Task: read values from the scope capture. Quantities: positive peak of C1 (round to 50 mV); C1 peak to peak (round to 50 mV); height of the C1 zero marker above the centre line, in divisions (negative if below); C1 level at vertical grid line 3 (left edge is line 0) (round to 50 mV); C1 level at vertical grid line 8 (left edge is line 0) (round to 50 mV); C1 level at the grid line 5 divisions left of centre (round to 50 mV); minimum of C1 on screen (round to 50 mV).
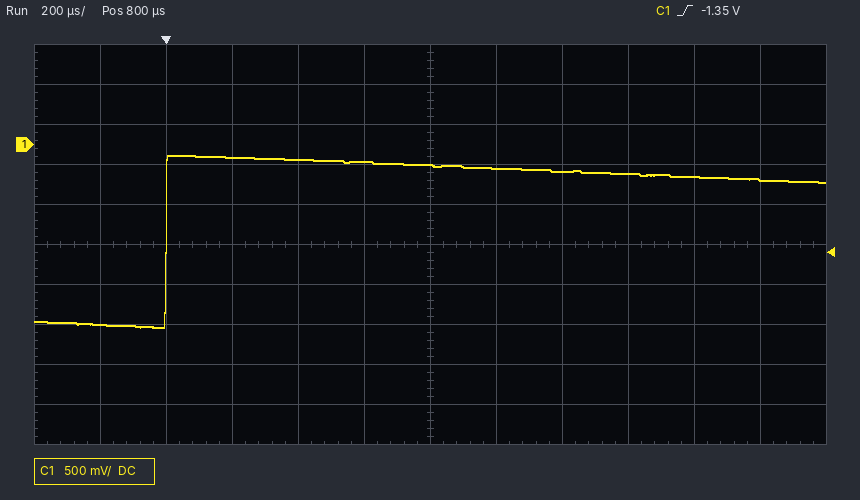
-150 mV
2.15 V
+2.5 div
-150 mV
-350 mV
-2.25 V
-2.30 V
